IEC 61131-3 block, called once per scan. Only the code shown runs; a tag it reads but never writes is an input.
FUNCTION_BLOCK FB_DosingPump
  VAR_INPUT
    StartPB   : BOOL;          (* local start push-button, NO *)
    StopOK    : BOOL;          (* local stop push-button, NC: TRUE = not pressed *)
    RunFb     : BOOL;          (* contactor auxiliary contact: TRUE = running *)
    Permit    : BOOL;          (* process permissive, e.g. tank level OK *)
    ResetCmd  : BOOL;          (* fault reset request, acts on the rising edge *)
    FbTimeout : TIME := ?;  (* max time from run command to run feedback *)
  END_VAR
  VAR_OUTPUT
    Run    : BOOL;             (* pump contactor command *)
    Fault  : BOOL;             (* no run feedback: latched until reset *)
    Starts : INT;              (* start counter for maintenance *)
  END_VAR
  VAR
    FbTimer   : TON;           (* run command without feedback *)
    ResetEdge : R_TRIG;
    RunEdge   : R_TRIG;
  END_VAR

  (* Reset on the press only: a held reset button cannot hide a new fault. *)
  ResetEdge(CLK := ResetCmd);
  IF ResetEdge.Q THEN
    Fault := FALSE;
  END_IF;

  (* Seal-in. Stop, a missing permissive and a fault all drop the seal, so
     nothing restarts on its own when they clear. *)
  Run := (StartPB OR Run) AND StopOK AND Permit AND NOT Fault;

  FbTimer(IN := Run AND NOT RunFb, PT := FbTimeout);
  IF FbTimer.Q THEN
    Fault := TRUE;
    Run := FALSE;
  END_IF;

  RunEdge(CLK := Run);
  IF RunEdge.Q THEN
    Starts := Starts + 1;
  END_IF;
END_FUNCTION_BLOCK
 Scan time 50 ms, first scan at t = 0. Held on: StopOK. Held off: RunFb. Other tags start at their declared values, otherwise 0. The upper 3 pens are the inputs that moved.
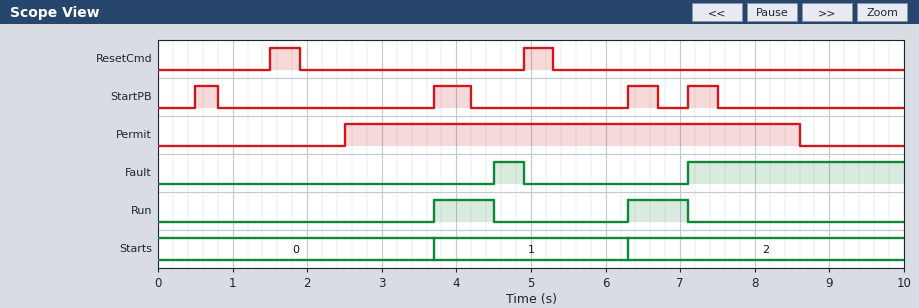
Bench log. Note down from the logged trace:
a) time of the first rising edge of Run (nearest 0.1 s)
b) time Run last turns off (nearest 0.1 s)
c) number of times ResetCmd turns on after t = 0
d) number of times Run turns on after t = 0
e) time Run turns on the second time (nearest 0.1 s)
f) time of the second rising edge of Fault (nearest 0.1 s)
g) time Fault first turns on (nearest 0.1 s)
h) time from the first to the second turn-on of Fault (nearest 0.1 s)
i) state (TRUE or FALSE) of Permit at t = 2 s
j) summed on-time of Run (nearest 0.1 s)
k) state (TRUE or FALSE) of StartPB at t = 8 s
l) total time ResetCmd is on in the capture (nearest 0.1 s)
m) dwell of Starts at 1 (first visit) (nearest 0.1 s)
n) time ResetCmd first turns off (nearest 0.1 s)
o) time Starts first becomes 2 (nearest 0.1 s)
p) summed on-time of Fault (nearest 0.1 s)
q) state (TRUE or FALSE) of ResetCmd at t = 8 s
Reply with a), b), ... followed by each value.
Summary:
a) 3.7 s
b) 7.1 s
c) 2
d) 2
e) 6.3 s
f) 7.1 s
g) 4.5 s
h) 2.6 s
i) FALSE
j) 1.6 s
k) FALSE
l) 0.8 s
m) 2.6 s
n) 1.9 s
o) 6.3 s
p) 3.3 s
q) FALSE
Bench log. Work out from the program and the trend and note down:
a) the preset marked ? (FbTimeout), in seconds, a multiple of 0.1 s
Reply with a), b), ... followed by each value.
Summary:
a) 0.8 s
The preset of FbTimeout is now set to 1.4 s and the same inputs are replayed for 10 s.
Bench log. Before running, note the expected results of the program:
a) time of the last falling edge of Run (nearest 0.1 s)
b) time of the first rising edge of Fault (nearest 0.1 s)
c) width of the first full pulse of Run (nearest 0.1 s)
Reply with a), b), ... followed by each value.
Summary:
a) 5.1 s
b) 5.1 s
c) 1.4 s
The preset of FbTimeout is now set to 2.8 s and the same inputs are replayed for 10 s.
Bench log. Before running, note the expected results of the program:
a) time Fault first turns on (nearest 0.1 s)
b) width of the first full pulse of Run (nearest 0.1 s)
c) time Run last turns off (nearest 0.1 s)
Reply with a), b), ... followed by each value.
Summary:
a) 6.5 s
b) 2.8 s
c) 6.5 s
